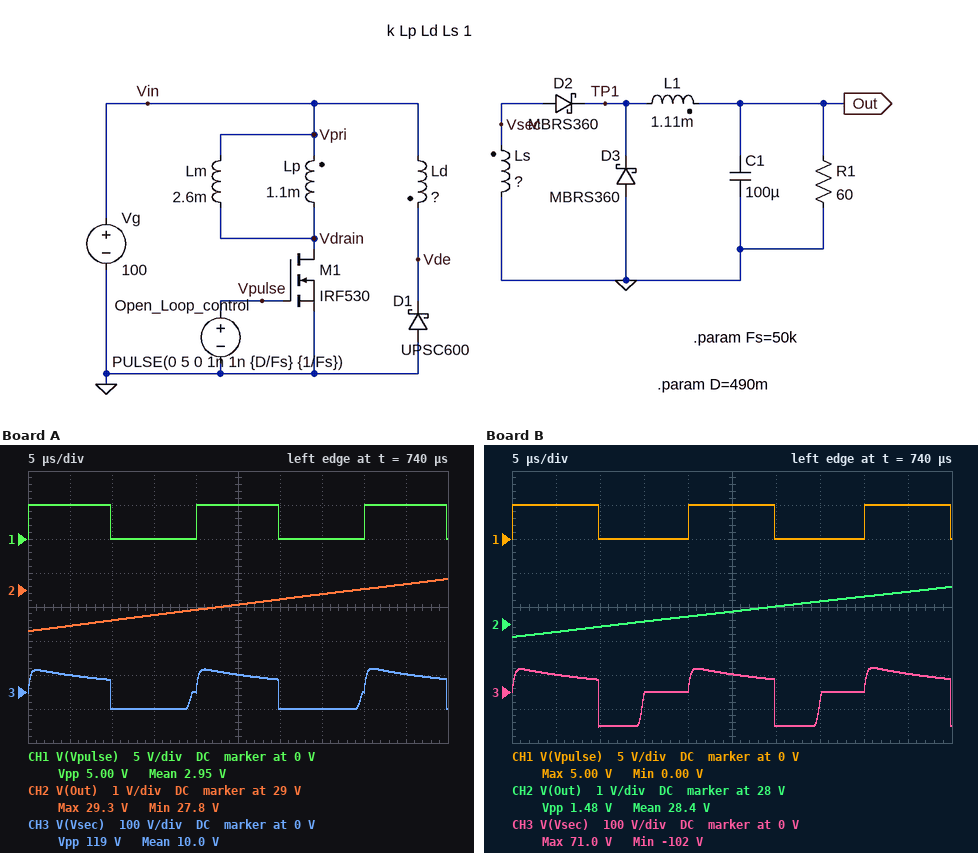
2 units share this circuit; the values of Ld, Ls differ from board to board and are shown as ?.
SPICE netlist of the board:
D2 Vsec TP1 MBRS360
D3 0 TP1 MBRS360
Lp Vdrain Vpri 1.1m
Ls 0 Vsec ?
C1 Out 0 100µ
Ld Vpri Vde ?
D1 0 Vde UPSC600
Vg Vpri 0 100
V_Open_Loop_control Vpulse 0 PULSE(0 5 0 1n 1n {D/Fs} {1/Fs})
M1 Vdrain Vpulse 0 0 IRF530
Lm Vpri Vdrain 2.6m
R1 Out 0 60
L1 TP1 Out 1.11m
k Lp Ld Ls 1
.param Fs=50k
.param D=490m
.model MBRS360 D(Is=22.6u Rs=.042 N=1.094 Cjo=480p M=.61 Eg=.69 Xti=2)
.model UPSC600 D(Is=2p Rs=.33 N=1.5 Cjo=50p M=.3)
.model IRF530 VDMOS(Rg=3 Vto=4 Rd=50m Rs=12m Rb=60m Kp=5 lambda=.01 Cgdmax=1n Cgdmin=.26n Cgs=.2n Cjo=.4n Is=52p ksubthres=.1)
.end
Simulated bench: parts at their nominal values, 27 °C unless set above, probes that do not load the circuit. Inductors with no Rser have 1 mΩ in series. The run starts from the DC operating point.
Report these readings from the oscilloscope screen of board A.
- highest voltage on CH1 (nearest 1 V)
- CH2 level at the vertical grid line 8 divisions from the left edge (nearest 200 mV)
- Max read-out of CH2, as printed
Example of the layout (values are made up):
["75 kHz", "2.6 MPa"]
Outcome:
["5 V", "29.0 V", "29.3 V"]
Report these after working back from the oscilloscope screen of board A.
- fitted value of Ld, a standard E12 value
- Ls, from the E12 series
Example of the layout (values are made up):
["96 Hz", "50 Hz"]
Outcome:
["2.2 mH", "560 µH"]
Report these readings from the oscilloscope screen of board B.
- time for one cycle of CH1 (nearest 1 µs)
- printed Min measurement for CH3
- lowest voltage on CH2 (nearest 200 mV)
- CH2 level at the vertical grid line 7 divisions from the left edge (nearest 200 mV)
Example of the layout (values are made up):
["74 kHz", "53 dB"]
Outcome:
["20 µs", "-102 V", "27.6 V", "28.6 V"]
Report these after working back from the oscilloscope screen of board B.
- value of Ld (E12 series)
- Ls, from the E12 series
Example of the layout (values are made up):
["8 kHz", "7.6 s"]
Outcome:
["680 µH", "680 µH"]
